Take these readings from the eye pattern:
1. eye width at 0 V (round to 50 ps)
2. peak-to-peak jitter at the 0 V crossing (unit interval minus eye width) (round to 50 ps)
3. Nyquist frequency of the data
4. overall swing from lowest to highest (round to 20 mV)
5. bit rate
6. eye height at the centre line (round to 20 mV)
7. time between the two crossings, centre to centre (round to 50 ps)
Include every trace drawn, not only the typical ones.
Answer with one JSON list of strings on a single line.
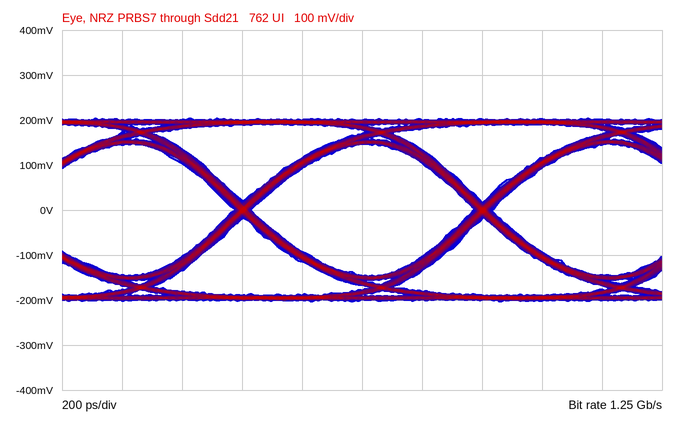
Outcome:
["750 ps", "50 ps", "625 MHz", "400 mV", "1.25 Gb/s", "300 mV", "800 ps"]
